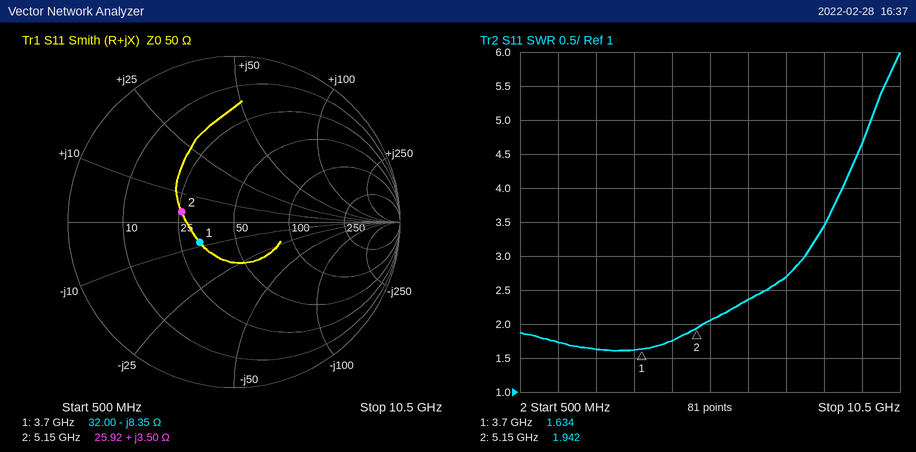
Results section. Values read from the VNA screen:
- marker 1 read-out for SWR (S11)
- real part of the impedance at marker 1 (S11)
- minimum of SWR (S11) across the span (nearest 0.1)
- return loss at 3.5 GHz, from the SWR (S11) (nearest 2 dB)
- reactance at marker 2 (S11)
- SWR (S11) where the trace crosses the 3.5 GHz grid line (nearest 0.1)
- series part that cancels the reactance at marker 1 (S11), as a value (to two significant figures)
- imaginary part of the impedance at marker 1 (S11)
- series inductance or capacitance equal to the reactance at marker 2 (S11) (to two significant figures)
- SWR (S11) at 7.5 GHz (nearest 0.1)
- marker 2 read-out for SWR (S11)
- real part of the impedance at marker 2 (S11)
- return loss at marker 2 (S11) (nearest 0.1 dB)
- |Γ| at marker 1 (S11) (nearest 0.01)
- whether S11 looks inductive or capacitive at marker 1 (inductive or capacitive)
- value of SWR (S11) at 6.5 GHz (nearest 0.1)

1.634
32.00 Ω
1.6
12 dB
+3.50 Ω
1.6
360 pH
-8.35 Ω
110 pH
2.7
1.942
25.92 Ω
9.9 dB
0.24
capacitive
2.4
